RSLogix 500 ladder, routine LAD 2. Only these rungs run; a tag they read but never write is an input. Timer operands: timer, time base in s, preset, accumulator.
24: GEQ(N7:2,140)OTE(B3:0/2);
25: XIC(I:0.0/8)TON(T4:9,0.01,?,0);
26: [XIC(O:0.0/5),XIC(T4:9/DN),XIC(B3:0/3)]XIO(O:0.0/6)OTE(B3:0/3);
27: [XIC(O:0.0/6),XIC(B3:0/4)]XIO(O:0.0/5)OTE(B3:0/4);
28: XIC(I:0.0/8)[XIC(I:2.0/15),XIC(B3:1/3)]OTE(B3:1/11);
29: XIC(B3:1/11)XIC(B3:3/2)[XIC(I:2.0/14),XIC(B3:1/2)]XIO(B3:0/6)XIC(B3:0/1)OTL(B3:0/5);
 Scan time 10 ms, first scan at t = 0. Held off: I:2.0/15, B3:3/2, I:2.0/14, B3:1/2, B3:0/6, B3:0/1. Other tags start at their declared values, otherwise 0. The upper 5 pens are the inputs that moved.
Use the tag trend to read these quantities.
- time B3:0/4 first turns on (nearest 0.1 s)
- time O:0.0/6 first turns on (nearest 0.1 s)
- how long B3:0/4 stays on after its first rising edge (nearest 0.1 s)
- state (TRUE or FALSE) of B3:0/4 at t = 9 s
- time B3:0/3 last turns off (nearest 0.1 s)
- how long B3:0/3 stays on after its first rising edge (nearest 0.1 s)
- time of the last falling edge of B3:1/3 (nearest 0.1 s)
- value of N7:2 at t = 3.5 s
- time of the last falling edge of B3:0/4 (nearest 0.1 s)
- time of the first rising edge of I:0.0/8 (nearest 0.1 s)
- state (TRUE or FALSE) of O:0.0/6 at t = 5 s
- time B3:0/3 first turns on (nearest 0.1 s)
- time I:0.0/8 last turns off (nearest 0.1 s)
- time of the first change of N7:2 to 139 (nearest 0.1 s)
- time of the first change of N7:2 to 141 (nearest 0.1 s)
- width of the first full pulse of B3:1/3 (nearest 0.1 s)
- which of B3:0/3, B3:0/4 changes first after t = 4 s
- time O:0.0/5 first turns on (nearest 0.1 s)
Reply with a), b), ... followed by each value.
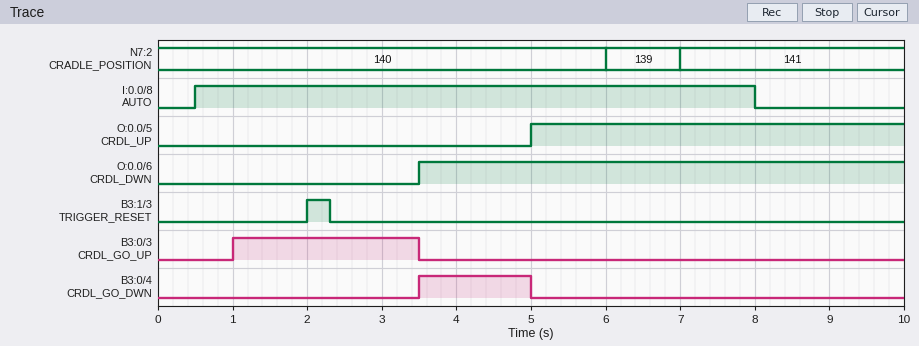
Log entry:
a) 3.5 s
b) 3.5 s
c) 1.5 s
d) FALSE
e) 3.5 s
f) 2.5 s
g) 2.3 s
h) 140
i) 5.0 s
j) 0.5 s
k) TRUE
l) 1.0 s
m) 8.0 s
n) 6.0 s
o) 7.0 s
p) 0.3 s
q) B3:0/4
r) 5.0 s
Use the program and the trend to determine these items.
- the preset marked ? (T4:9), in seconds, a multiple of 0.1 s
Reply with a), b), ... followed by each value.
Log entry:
a) 0.5 s
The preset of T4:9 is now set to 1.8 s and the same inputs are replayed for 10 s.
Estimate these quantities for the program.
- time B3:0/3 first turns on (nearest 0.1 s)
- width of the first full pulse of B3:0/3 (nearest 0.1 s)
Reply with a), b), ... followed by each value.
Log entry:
a) 2.3 s
b) 1.2 s
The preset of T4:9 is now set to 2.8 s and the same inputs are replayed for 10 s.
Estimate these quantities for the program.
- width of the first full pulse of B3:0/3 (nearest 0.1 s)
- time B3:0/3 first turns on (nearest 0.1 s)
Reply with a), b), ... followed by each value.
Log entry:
a) 0.2 s
b) 3.3 s
